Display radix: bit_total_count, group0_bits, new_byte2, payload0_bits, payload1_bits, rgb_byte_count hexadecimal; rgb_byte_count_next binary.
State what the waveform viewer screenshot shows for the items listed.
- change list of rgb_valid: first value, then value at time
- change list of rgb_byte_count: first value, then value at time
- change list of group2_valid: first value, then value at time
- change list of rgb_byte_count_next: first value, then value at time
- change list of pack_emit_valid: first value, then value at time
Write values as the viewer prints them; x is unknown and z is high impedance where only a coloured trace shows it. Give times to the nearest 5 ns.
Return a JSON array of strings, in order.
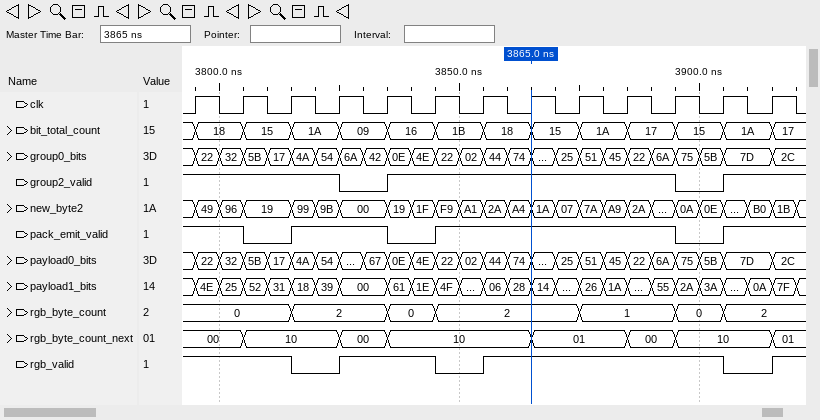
["1, 0 at 3815 ns, 1 at 3825 ns, 0 at 3845 ns, 1 at 3855 ns, 0 at 3905 ns, 1 at 3915 ns", "0, 2 at 3815 ns, 0 at 3835 ns, 2 at 3845 ns, 1 at 3875 ns, 0 at 3895 ns, 2 at 3905 ns", "1, 0 at 3825 ns, 1 at 3835 ns, 0 at 3895 ns, 1 at 3905 ns", "00, 10 at 3805 ns, 00 at 3825 ns, 10 at 3835 ns, 01 at 3865 ns, 00 at 3885 ns, 10 at 3895 ns, 01 at 3915 ns", "1, 0 at 3805 ns, 1 at 3815 ns, 0 at 3835 ns, 1 at 3845 ns, 0 at 3895 ns, 1 at 3905 ns"]
